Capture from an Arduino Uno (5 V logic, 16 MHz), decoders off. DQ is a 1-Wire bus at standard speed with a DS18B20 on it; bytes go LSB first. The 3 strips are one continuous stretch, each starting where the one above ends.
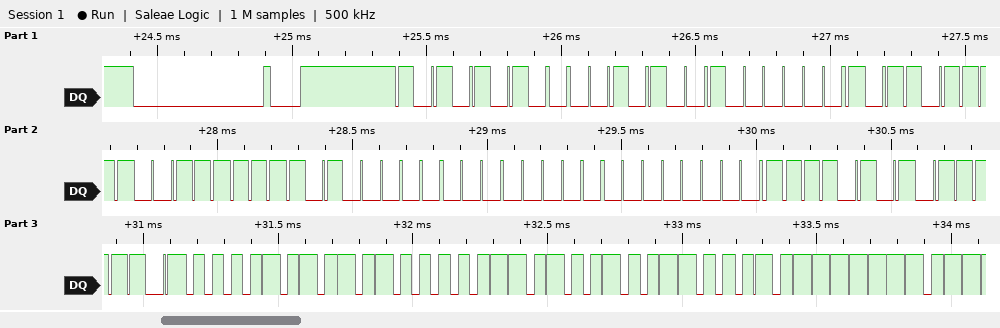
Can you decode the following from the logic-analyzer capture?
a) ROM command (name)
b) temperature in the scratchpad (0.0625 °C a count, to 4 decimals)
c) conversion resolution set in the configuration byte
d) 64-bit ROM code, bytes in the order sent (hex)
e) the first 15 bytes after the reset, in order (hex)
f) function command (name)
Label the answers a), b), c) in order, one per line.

a) Match ROM
b) 85.0000 °C
c) 12 bits
d) 28 81 F6 FC 05 00 00 AF
e) 55 28 81 F6 FC 05 00 00 AF BE 50 05 4B 46 7F
f) Read Scratchpad
